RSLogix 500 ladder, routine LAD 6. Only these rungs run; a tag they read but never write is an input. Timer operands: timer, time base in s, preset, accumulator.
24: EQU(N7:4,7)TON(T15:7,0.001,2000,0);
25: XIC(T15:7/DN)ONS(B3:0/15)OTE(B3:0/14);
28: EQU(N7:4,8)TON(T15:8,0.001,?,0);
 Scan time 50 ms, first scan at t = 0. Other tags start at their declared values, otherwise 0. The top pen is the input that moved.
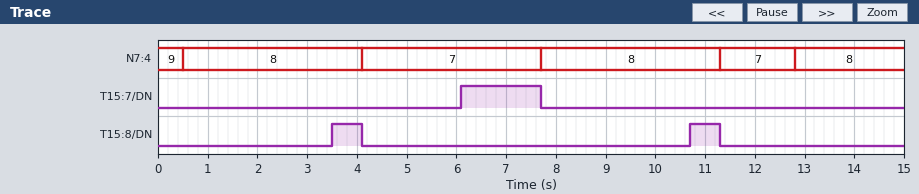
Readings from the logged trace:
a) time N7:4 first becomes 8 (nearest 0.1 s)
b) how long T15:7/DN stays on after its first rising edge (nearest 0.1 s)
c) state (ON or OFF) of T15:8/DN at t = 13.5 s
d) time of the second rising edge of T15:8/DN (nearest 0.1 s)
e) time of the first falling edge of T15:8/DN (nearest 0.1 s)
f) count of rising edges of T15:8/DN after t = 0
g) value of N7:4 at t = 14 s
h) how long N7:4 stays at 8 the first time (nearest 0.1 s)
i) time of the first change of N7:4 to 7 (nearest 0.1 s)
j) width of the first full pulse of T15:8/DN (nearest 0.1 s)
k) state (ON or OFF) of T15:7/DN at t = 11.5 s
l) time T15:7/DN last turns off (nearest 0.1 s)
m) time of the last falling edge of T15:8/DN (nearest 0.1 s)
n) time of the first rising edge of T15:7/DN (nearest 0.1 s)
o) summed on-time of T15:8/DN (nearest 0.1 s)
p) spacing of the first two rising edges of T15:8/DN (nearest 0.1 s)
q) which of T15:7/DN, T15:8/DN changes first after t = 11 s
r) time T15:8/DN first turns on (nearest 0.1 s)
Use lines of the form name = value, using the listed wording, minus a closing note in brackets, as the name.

time N7:4 first becomes 8 = 0.5 s
how long T15:7/DN stays on after its first rising edge = 1.6 s
state (ON or OFF) of T15:8/DN at t = 13.5 s = OFF
time of the second rising edge of T15:8/DN = 10.7 s
time of the first falling edge of T15:8/DN = 4.1 s
count of rising edges of T15:8/DN after t = 0 = 2
value of N7:4 at t = 14 s = 8
how long N7:4 stays at 8 the first time = 3.6 s
time of the first change of N7:4 to 7 = 4.1 s
width of the first full pulse of T15:8/DN = 0.6 s
state (ON or OFF) of T15:7/DN at t = 11.5 s = OFF
time T15:7/DN last turns off = 7.7 s
time of the last falling edge of T15:8/DN = 11.3 s
time of the first rising edge of T15:7/DN = 6.1 s
summed on-time of T15:8/DN = 1.2 s
spacing of the first two rising edges of T15:8/DN = 7.2 s
which of T15:7/DN, T15:8/DN changes first after t = 11 s = T15:8/DN
time T15:8/DN first turns on = 3.5 s
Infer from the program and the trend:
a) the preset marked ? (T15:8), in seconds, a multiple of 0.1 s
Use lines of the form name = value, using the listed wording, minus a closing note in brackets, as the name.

the preset marked ? (T15:8), in seconds, a multiple of 0.1 s = 3.0 s
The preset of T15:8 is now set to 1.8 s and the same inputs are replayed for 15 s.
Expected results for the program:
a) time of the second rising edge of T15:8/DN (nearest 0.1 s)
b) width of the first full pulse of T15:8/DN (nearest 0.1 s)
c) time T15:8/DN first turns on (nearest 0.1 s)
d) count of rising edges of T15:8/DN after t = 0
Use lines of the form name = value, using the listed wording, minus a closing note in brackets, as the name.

time of the second rising edge of T15:8/DN = 9.5 s
width of the first full pulse of T15:8/DN = 1.8 s
time T15:8/DN first turns on = 2.3 s
count of rising edges of T15:8/DN after t = 0 = 3
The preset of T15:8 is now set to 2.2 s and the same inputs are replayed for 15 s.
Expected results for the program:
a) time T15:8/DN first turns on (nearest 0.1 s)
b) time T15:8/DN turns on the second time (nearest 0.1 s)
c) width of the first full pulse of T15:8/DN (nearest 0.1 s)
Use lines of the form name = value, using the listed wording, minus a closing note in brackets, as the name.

time T15:8/DN first turns on = 2.7 s
time T15:8/DN turns on the second time = 9.9 s
width of the first full pulse of T15:8/DN = 1.4 s
